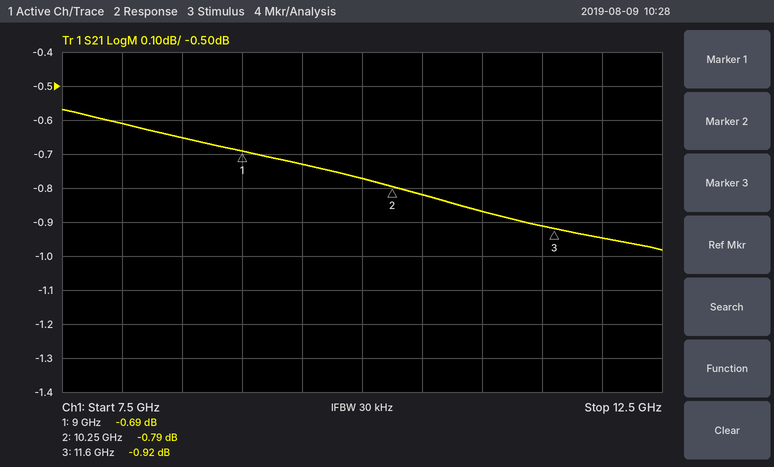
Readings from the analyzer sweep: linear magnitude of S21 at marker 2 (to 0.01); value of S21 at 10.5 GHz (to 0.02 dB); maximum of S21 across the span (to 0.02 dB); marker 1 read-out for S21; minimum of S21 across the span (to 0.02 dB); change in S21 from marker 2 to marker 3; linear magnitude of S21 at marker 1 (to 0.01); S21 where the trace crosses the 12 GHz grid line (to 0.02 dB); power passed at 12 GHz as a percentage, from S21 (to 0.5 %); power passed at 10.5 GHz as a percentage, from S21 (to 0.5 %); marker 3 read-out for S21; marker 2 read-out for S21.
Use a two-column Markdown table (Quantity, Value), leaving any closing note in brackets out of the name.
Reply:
| Quantity | Value |
|---|---|
| linear magnitude of S21 at marker 2 | 0.91 |
| value of S21 at 10.5 GHz | -0.82 dB |
| maximum of S21 across the span | -0.56 dB |
| marker 1 read-out for S21 | -0.69 dB |
| minimum of S21 across the span | -0.98 dB |
| change in S21 from marker 2 to marker 3 | -0.13 dB |
| linear magnitude of S21 at marker 1 | 0.92 |
| S21 where the trace crosses the 12 GHz grid line | -0.94 dB |
| power passed at 12 GHz as a percentage, from S21 | 80.5 % |
| power passed at 10.5 GHz as a percentage, from S21 | 83.0 % |
| marker 3 read-out for S21 | -0.92 dB |
| marker 2 read-out for S21 | -0.79 dB |
